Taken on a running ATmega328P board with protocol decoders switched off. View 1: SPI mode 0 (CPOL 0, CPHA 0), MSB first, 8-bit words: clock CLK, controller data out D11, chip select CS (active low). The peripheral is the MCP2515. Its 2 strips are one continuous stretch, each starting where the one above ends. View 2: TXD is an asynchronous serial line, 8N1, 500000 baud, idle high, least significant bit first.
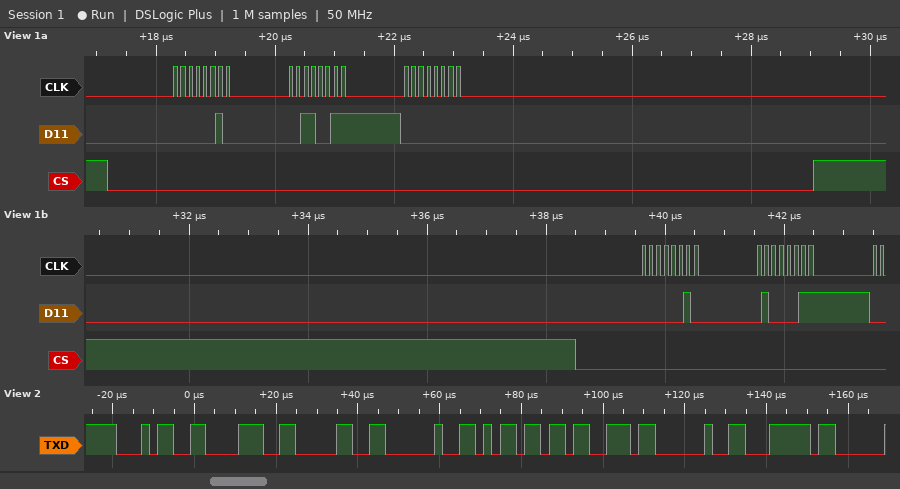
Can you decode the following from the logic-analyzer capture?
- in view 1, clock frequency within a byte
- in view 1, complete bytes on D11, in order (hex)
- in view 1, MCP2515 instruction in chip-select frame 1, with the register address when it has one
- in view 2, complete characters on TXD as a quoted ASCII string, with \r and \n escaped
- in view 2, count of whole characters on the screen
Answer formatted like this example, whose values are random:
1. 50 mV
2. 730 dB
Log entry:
1. 8 MHz
2. 02 33 00 02 43
3. WRITE 0x33
4. "480 ms |"
5. 8
